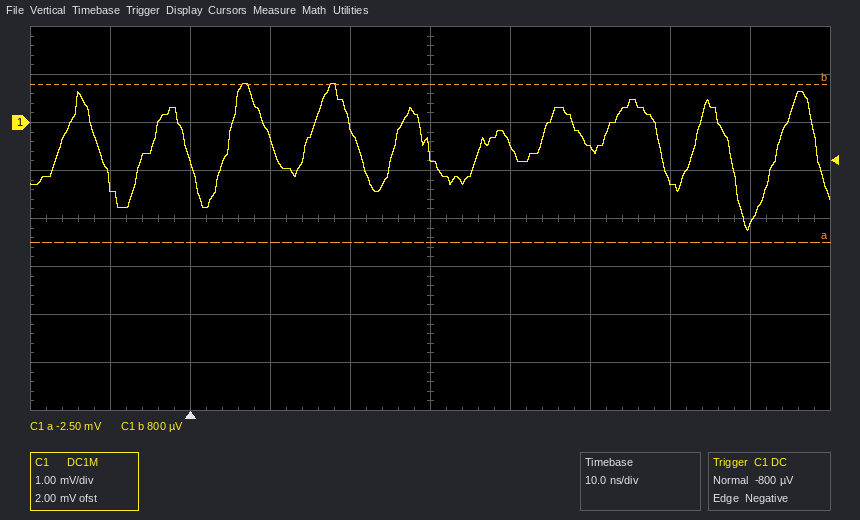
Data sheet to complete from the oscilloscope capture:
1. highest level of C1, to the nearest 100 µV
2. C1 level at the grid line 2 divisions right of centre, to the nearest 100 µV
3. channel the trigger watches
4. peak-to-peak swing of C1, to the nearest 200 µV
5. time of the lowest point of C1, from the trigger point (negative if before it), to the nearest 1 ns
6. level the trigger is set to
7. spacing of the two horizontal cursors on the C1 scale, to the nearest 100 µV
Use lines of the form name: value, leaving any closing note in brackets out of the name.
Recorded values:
highest level of C1, to the nearest 100 µV: 800 µV
C1 level at the grid line 2 divisions right of centre, to the nearest 100 µV: -500 µV
channel the trigger watches: C1
peak-to-peak swing of C1, to the nearest 200 µV: 3.0 mV
time of the lowest point of C1, from the trigger point (negative if before it), to the nearest 1 ns: +70 ns
level the trigger is set to: -800 µV
spacing of the two horizontal cursors on the C1 scale, to the nearest 100 µV: 3.3 mV
